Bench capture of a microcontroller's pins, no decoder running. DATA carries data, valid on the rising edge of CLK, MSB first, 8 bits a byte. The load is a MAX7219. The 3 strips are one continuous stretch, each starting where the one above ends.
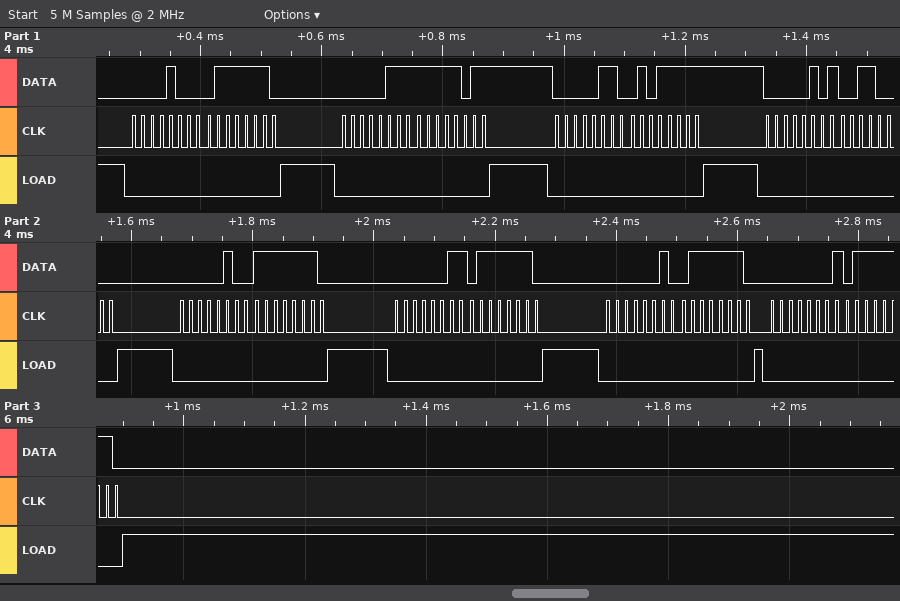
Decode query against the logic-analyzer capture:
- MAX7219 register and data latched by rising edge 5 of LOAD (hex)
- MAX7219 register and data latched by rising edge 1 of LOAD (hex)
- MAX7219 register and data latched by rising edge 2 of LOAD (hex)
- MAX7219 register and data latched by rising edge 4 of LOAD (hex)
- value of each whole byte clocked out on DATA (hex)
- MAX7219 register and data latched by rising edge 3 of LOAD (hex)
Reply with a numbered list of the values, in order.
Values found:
1. register 0x4, data 0xFE
2. register 0x8, data 0x7E
3. register 0x7, data 0xFB
4. register 0x5, data 0x30
5. 08 7E 07 FB 06 5F 05 30 04 FE 03 7E 02 7E 01 7E
6. register 0x6, data 0x5F
